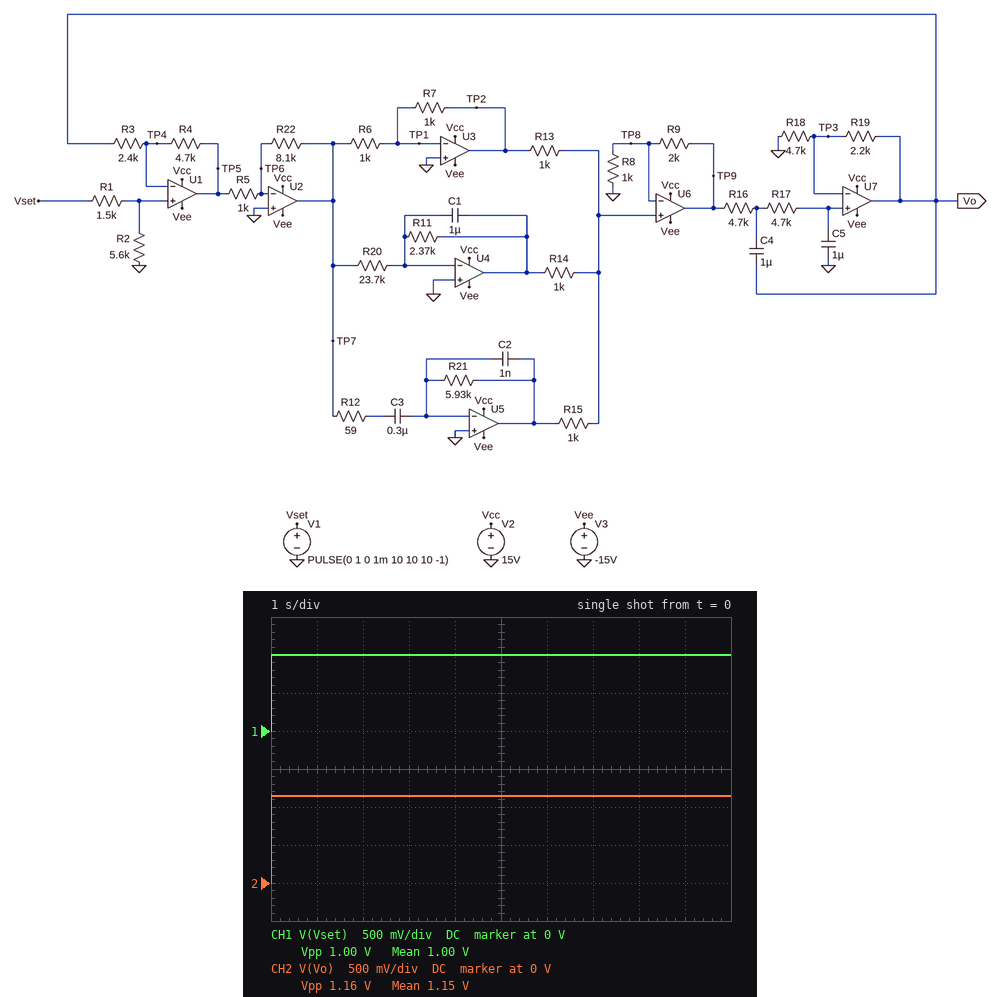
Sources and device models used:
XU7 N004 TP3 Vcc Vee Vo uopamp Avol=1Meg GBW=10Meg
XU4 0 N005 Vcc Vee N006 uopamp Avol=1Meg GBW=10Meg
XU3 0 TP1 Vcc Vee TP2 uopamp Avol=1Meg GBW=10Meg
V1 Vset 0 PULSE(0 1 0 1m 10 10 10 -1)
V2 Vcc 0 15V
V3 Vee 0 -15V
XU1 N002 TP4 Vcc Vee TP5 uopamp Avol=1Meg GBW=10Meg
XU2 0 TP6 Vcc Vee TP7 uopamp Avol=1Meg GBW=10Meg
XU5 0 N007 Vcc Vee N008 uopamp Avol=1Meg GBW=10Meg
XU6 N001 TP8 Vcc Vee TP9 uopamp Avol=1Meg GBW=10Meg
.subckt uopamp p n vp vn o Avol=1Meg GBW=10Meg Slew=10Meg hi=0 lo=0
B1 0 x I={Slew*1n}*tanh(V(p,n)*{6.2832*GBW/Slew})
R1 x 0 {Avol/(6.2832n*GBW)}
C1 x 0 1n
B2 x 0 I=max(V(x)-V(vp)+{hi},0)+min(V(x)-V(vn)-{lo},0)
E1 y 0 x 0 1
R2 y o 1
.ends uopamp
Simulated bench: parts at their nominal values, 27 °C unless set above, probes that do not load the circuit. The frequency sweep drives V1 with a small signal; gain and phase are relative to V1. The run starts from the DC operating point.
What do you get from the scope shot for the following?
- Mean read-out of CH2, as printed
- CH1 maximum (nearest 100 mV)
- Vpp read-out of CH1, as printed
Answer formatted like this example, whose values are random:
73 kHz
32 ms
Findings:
1.15 V
1.0 V
1.00 V
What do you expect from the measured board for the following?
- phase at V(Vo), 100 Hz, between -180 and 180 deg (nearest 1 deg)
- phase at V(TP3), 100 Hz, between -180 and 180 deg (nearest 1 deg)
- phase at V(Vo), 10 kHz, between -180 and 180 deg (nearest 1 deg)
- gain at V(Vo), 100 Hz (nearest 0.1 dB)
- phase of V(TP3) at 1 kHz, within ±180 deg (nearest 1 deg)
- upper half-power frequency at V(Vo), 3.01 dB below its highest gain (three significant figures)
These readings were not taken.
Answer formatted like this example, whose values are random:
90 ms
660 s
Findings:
-15 deg
-15 deg
-164 deg
1.8 dB
-83 deg
343 Hz
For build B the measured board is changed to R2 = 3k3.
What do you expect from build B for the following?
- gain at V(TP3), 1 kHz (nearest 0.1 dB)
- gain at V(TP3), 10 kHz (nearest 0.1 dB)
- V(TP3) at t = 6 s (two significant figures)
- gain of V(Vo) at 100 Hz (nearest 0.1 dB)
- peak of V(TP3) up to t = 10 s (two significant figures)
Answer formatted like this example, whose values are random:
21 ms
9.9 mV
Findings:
-13.3 dB
-37.1 dB
680 mV
0.6 dB
690 mV
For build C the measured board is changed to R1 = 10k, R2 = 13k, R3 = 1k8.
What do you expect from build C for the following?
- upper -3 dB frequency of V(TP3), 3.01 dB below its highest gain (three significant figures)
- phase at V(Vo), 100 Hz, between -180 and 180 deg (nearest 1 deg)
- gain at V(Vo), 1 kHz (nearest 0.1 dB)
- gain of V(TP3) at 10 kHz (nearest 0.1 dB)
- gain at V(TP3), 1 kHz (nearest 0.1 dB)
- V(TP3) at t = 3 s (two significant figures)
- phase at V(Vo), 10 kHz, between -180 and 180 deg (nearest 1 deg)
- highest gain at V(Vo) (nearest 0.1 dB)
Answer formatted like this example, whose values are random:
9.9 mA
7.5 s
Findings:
449 Hz
-11 deg
-10.1 dB
-37.0 dB
-13.4 dB
520 mV
-164 deg
-1.9 dB
